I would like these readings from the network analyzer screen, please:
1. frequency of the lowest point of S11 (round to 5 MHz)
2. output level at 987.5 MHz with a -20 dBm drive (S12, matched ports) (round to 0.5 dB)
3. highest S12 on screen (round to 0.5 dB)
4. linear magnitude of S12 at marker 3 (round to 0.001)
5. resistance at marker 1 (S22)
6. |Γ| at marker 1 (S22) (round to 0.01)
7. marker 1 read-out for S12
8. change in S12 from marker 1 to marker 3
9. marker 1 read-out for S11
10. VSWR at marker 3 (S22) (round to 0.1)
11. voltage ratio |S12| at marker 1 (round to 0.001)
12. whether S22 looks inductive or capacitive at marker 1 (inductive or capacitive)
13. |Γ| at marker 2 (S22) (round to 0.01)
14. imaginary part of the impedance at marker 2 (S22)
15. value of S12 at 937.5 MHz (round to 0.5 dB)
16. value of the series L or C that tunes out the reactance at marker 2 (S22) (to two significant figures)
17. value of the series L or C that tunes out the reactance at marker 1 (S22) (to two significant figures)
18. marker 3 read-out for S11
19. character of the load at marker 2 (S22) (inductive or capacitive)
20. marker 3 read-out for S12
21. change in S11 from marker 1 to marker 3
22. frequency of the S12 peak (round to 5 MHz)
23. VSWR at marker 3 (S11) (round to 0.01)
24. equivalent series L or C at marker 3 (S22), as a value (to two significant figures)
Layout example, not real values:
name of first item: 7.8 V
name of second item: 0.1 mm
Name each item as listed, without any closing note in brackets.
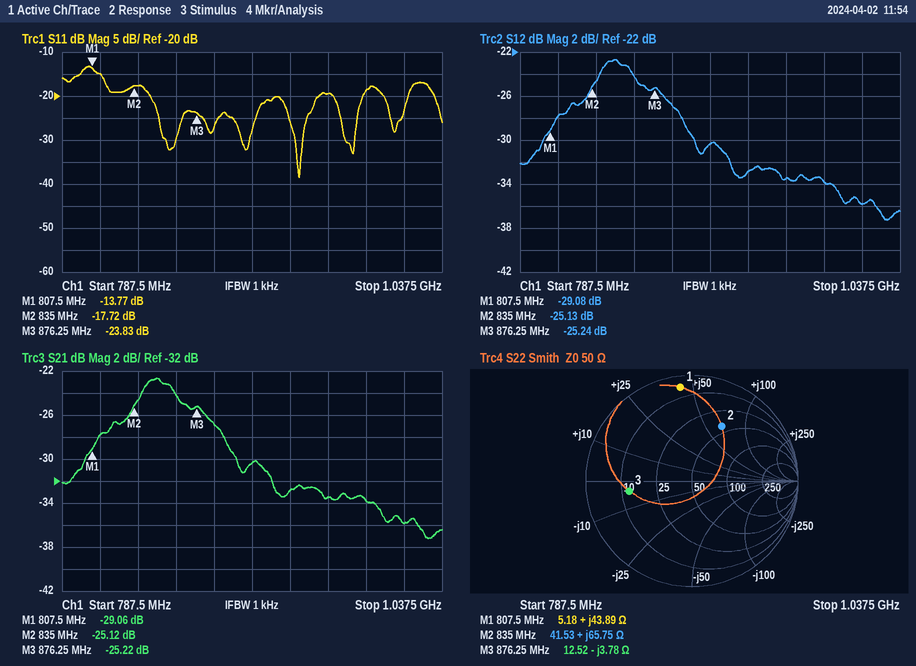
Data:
frequency of the lowest point of S11: 945 MHz
output level at 987.5 MHz with a -20 dBm drive (S12, matched ports): -54.0 dBm
highest S12 on screen: -22.5 dB
linear magnitude of S12 at marker 3: 0.055
resistance at marker 1: 5.18 Ω
|Γ| at marker 1 (S22): 0.89
marker 1 read-out for S12: -29.08 dB
change in S12 from marker 1 to marker 3: 3.84 dB
marker 1 read-out for S11: -13.77 dB
VSWR at marker 3 (S22): 4.0
voltage ratio |S12| at marker 1: 0.035
whether S22 looks inductive or capacitive at marker 1: inductive
|Γ| at marker 2 (S22): 0.59
imaginary part of the impedance at marker 2: +65.75 Ω
value of S12 at 937.5 MHz: -33.0 dB
value of the series L or C that tunes out the reactance at marker 2 (S22): 2.9 pF
value of the series L or C that tunes out the reactance at marker 1 (S22): 4.5 pF
marker 3 read-out for S11: -23.83 dB
character of the load at marker 2 (S22): inductive
marker 3 read-out for S12: -25.24 dB
change in S11 from marker 1 to marker 3: -10.06 dB
frequency of the S12 peak: 850 MHz
VSWR at marker 3 (S11): 1.14
equivalent series L or C at marker 3 (S22), as a value: 48 pF
